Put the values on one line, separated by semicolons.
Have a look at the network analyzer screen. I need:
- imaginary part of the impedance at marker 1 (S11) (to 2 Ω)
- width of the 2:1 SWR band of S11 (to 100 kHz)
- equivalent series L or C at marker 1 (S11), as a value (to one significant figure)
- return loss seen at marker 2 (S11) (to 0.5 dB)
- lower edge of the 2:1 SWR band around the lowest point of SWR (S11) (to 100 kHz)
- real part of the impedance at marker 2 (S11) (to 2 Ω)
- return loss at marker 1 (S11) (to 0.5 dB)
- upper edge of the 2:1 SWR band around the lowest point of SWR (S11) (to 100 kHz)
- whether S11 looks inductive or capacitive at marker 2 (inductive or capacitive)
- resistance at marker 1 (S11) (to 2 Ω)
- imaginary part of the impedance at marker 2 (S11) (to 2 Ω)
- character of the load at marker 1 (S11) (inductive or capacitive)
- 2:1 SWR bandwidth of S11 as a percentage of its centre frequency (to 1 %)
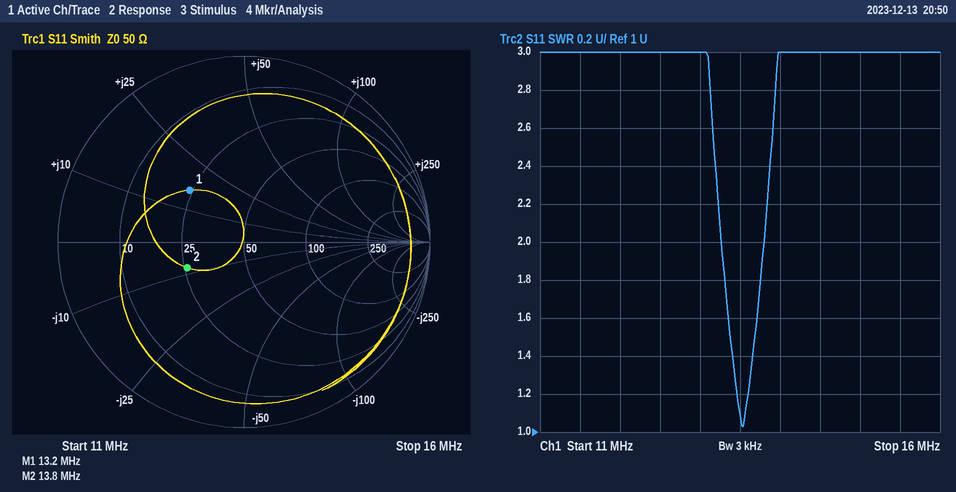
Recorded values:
+16 Ω; 500 kHz; 200 nH; 9.5 dB; 13.3 MHz; 26 Ω; 8.0 dB; 13.8 MHz; capacitive; 24 Ω; -8 Ω; inductive; 4 %
